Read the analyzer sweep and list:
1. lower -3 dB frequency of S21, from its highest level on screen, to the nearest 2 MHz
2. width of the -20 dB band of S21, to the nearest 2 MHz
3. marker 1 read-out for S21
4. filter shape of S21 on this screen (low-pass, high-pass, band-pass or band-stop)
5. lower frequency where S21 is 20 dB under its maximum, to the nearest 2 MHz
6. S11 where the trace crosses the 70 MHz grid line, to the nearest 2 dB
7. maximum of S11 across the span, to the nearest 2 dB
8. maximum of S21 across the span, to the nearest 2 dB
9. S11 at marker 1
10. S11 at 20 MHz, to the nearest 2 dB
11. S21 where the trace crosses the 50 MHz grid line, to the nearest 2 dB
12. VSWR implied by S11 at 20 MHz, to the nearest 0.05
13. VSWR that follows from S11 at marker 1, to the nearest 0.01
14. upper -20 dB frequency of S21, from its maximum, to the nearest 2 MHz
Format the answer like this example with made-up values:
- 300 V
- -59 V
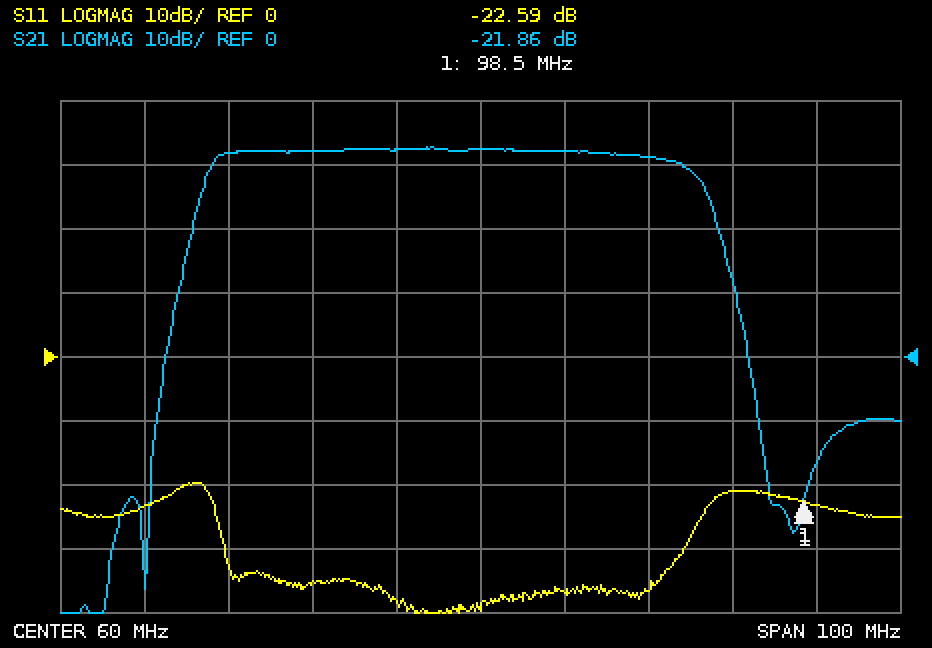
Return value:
- 28 MHz
- 66 MHz
- -21.86 dB
- band-pass
- 24 MHz
- -36 dB
- -20 dB
- 32 dB
- -22.59 dB
- -24 dB
- 32 dB
- 1.15
- 1.16
- 90 MHz
